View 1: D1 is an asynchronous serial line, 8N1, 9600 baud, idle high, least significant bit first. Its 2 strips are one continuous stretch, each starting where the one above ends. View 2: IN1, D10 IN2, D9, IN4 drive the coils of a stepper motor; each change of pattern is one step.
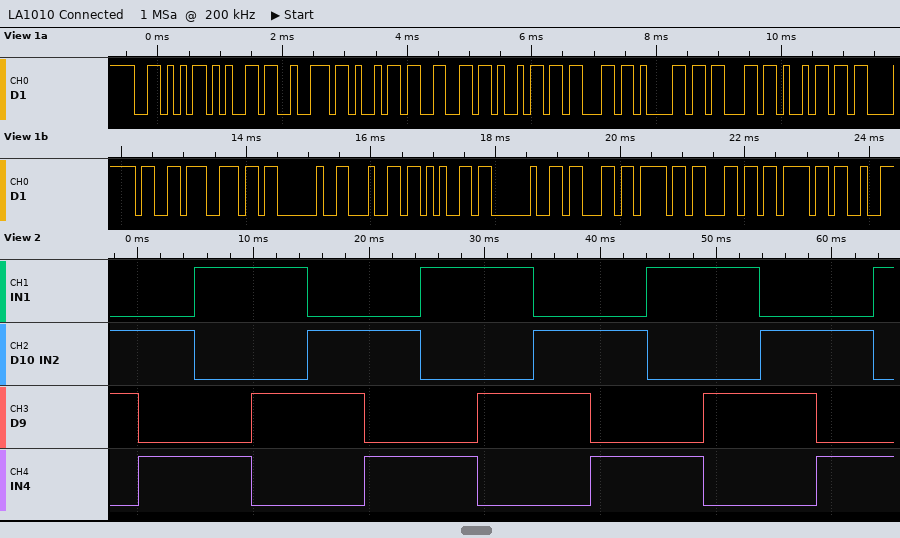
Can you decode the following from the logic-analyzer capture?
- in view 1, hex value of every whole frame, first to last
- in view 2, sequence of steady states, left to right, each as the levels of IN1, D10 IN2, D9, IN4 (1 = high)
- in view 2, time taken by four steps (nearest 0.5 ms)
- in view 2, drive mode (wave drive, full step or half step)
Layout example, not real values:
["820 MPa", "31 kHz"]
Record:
["56 65 72 69 66 69 63 61 63 69 C3 B3 6E 20 64 65 20 63 6F 6C 6F", "0110 0101 1001 1010 0110 0101 1001 1010 0110 0101 1001 1010 0110 0101 1001", "19.5 ms", "full step"]
